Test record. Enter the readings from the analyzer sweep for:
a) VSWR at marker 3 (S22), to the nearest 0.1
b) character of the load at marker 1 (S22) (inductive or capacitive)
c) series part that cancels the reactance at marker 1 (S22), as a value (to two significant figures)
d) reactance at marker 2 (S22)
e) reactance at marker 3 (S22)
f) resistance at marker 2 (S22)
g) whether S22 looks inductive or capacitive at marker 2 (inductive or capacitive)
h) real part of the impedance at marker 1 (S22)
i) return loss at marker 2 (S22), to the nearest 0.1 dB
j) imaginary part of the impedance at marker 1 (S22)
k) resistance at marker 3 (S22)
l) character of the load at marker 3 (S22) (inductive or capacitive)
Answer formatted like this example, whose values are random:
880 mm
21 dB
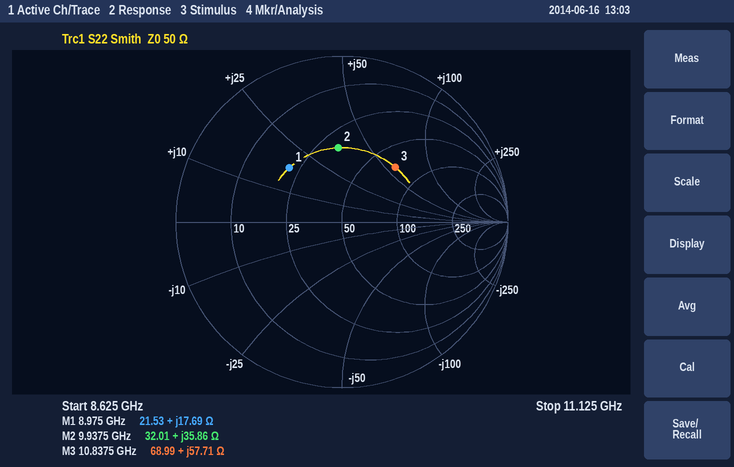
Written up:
2.7
inductive
1.0 pF
+35.86 Ω
+57.71 Ω
32.01 Ω
inductive
21.53 Ω
7.0 dB
+17.69 Ω
68.99 Ω
inductive
